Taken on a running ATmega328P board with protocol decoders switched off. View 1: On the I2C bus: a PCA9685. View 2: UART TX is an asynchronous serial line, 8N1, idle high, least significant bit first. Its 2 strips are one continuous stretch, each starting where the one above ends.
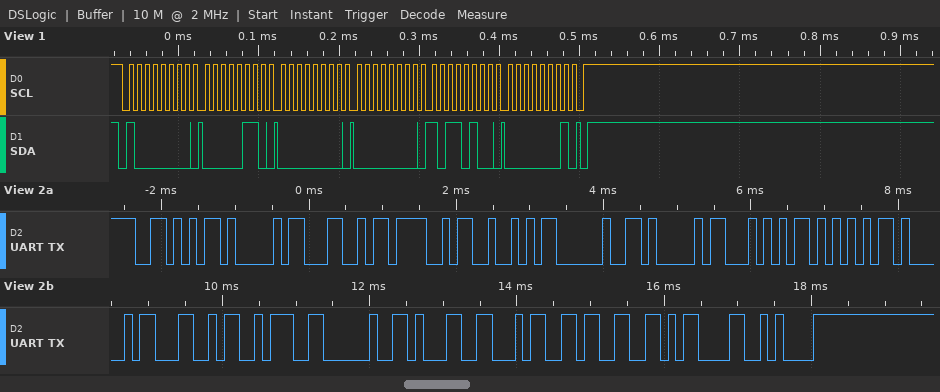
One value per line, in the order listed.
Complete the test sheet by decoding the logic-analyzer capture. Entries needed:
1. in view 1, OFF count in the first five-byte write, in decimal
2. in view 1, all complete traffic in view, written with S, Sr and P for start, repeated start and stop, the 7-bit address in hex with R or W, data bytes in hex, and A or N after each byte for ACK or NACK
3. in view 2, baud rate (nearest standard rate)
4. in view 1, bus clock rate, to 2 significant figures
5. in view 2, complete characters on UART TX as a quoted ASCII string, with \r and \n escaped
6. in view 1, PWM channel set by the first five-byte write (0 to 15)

436
S 40W A 06 A 00 A 00 A B4 A 01 A P
9600 baud
100 kHz
"VALOR ATUAL: 143\r\n"
0
